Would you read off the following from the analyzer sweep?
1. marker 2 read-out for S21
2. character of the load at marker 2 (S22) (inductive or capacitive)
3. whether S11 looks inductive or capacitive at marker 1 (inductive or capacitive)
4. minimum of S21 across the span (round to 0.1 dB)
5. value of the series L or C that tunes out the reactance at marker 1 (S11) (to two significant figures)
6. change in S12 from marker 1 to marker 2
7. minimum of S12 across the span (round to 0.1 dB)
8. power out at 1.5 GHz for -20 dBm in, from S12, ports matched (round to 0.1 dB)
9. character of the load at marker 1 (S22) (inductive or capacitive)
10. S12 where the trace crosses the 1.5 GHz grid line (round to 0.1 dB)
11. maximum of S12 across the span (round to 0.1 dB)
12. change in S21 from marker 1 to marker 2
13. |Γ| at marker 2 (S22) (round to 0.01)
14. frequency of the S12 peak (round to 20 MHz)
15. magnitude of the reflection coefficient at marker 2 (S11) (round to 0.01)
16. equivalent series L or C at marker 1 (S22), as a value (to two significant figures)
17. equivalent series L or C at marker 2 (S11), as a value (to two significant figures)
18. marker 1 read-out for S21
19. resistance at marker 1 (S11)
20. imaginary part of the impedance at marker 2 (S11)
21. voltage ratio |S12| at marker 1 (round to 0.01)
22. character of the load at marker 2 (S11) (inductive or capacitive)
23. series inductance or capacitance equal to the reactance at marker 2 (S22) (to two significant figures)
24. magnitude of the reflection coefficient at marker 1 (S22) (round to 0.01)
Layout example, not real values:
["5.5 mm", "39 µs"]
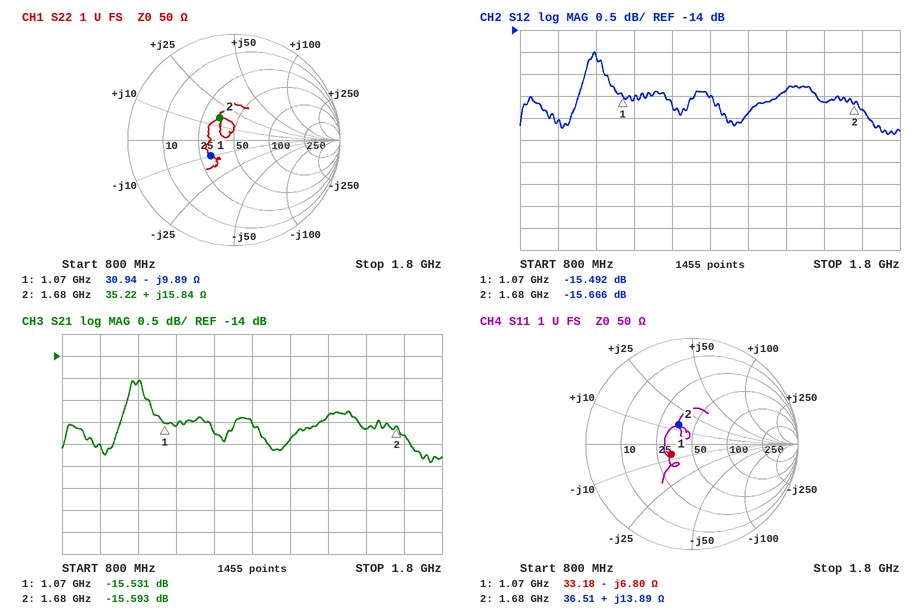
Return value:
["-15.593 dB", "inductive", "capacitive", "-16.4 dB", "1.0 nH", "-0.174 dB", "-16.4 dB", "-35.4 dBm", "capacitive", "-15.4 dB", "-14.5 dB", "-0.062 dB", "0.25", "1.00 GHz", "0.22", "15 pF", "1.3 nH", "-15.531 dB", "33.18 Ω", "+13.89 Ω", "0.17", "inductive", "1.5 nH", "0.26"]
